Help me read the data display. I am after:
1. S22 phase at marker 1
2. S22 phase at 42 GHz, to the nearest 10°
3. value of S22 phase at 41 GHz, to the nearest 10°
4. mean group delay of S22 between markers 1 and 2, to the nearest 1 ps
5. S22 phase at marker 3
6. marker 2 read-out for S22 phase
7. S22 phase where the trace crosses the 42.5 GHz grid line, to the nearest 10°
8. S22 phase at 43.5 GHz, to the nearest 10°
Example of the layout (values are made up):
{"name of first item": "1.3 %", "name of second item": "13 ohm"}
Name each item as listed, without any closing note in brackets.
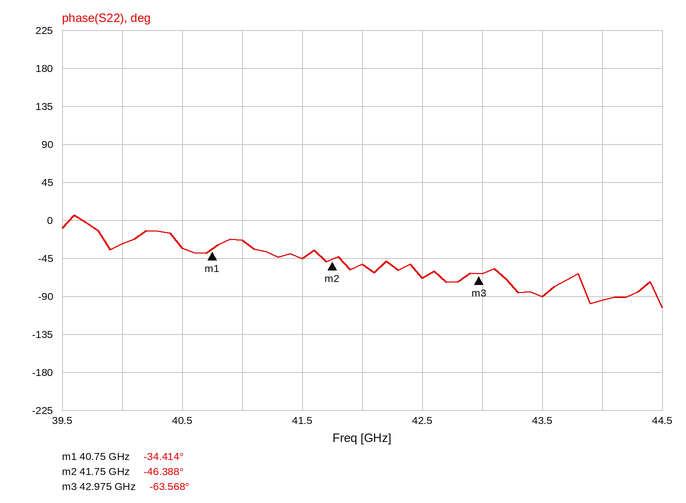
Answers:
{"S22 phase at marker 1": "-34.414°", "S22 phase at 42 GHz, to the nearest 10°": "-50°", "value of S22 phase at 41 GHz, to the nearest 10°": "-20°", "mean group delay of S22 between markers 1 and 2, to the nearest 1 ps": "33 ps", "S22 phase at marker 3": "-63.568°", "marker 2 read-out for S22 phase": "-46.388°", "S22 phase where the trace crosses the 42.5 GHz grid line, to the nearest 10°": "-70°", "S22 phase at 43.5 GHz, to the nearest 10°": "-90°"}
